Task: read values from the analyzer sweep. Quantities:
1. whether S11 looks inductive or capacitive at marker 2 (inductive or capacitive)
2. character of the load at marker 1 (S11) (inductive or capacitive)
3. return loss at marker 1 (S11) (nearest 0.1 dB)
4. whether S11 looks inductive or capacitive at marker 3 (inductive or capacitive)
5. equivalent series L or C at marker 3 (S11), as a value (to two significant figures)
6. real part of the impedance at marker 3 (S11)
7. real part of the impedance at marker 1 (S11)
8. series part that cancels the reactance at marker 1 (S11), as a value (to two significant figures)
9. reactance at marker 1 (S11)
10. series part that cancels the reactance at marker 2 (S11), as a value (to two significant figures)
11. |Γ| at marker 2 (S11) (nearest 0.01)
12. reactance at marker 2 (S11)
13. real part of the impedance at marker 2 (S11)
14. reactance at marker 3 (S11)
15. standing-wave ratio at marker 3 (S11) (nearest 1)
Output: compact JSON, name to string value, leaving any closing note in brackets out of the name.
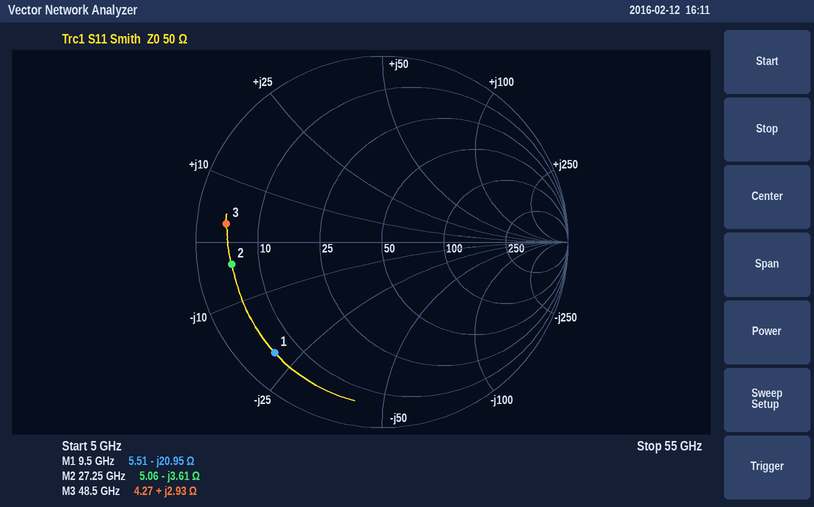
{"whether S11 looks inductive or capacitive at marker 2": "capacitive", "character of the load at marker 1 (S11)": "capacitive", "return loss at marker 1 (S11)": "1.6 dB", "whether S11 looks inductive or capacitive at marker 3": "inductive", "equivalent series L or C at marker 3 (S11), as a value": "9.6 pH", "real part of the impedance at marker 3": "4.27 Ω", "real part of the impedance at marker 1": "5.51 Ω", "series part that cancels the reactance at marker 1 (S11), as a value": "350 pH", "reactance at marker 1": "-20.95 Ω", "series part that cancels the reactance at marker 2 (S11), as a value": "21 pH", "|Γ| at marker 2 (S11)": "0.82", "reactance at marker 2": "-3.61 Ω", "real part of the impedance at marker 2": "5.06 Ω", "reactance at marker 3": "+2.93 Ω", "standing-wave ratio at marker 3 (S11)": "12"}
